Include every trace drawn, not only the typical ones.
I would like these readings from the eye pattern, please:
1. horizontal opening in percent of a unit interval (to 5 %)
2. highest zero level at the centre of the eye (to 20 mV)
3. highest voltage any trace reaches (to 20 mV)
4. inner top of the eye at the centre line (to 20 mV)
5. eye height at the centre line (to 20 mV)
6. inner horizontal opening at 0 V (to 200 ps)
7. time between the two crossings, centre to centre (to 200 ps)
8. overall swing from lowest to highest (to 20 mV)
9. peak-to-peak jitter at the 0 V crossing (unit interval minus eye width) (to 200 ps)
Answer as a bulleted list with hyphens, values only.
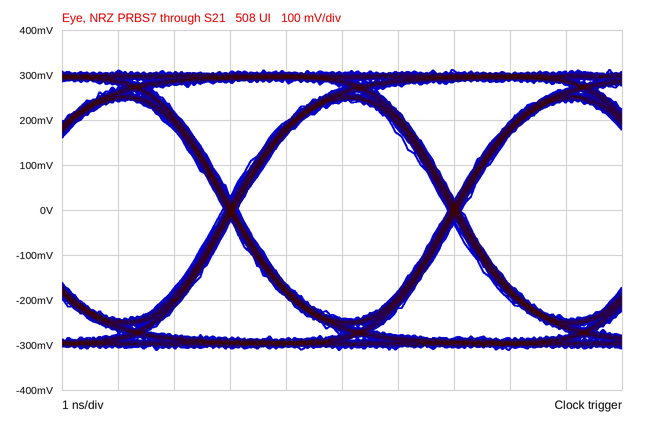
- 95 %
- -240 mV
- 320 mV
- 240 mV
- 480 mV
- 3.8 ns
- 4.0 ns
- 620 mV
- 200 ps
